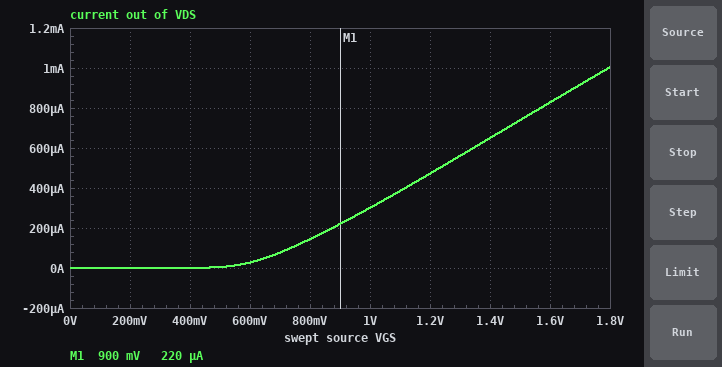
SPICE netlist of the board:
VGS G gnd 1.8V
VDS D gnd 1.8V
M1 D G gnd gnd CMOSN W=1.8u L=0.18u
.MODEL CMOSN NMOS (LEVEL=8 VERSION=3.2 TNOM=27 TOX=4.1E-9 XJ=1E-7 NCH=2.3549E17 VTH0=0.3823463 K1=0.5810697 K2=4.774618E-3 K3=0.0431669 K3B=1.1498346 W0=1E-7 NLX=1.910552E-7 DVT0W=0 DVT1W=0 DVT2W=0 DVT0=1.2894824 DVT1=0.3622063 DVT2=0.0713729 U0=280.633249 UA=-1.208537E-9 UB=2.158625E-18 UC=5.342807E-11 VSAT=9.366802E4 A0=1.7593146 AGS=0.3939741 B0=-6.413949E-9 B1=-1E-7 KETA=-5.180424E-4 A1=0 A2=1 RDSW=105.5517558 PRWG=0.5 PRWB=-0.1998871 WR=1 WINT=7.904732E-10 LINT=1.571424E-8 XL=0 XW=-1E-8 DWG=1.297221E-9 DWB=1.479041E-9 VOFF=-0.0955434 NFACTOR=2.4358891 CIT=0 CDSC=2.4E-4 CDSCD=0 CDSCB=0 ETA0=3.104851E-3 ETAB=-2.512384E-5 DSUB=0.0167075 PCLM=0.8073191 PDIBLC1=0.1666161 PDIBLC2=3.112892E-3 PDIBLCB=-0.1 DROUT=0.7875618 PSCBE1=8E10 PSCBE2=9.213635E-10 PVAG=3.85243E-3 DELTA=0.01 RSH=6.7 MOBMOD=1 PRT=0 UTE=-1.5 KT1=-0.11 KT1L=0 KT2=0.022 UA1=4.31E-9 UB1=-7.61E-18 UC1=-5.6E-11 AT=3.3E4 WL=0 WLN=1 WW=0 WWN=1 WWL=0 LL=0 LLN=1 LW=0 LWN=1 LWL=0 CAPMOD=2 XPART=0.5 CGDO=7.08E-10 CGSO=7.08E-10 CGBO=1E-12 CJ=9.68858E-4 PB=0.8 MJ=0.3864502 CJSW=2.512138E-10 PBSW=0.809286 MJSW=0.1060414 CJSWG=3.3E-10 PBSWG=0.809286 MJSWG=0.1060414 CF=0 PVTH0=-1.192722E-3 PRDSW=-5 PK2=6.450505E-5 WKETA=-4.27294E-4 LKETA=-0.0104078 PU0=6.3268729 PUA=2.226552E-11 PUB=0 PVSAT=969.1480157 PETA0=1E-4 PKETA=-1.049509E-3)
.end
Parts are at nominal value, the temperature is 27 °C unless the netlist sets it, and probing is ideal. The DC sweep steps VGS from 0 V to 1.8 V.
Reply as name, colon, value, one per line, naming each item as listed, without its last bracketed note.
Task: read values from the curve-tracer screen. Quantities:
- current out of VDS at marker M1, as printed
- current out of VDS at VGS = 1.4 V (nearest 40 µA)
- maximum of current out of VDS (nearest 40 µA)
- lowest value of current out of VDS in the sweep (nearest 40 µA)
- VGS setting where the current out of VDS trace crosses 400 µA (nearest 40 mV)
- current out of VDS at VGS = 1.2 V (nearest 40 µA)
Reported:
current out of VDS at marker M1, as printed: 220 µA
current out of VDS at VGS = 1.4 V: 640 µA
maximum of current out of VDS: 1.00 mA
lowest value of current out of VDS in the sweep: 0 A
VGS setting where the current out of VDS trace crosses 400 µA: 1.12 V
current out of VDS at VGS = 1.2 V: 480 µA
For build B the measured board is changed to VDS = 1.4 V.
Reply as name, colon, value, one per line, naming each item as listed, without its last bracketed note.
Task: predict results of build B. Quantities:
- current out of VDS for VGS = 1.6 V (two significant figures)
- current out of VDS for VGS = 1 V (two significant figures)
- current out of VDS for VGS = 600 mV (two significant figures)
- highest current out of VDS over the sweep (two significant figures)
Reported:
current out of VDS for VGS = 1.6 V: 810 µA
current out of VDS for VGS = 1 V: 290 µA
current out of VDS for VGS = 600 mV: 24 µA
highest current out of VDS over the sweep: 980 µA
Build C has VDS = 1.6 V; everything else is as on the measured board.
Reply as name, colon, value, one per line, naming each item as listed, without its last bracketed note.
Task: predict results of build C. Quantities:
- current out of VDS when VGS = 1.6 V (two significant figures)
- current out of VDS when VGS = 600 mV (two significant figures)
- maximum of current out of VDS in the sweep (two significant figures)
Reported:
current out of VDS when VGS = 1.6 V: 820 µA
current out of VDS when VGS = 600 mV: 26 µA
maximum of current out of VDS in the sweep: 990 µA
